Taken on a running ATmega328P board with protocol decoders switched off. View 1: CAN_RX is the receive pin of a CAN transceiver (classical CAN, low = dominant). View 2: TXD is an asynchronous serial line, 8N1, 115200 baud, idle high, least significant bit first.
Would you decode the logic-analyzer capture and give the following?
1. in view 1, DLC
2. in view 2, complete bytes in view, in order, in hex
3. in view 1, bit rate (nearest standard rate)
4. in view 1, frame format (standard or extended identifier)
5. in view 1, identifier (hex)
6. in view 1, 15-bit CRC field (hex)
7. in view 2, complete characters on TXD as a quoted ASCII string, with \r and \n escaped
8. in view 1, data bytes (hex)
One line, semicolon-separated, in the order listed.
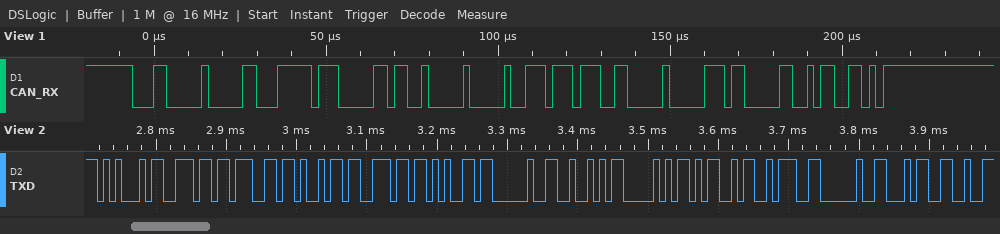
8; 45 6E 67 69 6E 65 20 52 50 4D 3A 20 34; 500 kbit/s; standard; 0x180; 0x0966; "Engine RPM: 4"; FF 05 90 00 EE E6 00 6C
